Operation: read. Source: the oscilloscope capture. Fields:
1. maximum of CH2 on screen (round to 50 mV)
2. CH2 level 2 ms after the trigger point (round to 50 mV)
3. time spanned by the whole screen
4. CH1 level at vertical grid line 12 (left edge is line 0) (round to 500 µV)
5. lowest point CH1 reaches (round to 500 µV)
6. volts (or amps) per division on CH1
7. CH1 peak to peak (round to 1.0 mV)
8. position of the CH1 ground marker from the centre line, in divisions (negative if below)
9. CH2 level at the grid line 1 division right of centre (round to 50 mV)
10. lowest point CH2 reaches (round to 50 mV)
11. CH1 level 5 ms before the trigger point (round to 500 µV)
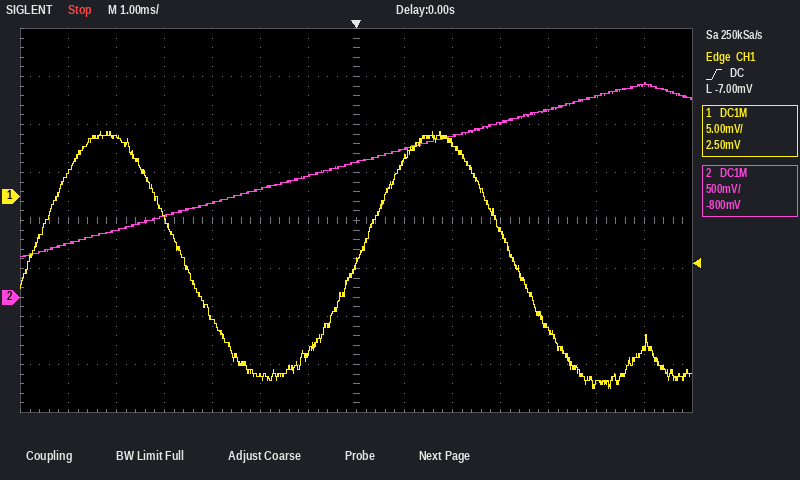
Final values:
2.25 V
1.70 V
14 ms
-19.5 mV
-20.0 mV
5 mV
27.0 mV
+0.5 div
1.55 V
400 mV
6.0 mV
